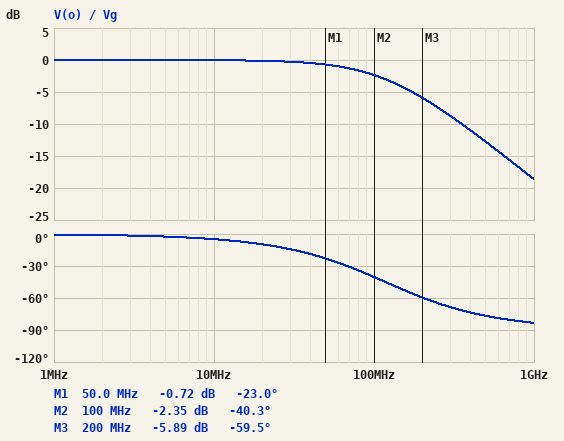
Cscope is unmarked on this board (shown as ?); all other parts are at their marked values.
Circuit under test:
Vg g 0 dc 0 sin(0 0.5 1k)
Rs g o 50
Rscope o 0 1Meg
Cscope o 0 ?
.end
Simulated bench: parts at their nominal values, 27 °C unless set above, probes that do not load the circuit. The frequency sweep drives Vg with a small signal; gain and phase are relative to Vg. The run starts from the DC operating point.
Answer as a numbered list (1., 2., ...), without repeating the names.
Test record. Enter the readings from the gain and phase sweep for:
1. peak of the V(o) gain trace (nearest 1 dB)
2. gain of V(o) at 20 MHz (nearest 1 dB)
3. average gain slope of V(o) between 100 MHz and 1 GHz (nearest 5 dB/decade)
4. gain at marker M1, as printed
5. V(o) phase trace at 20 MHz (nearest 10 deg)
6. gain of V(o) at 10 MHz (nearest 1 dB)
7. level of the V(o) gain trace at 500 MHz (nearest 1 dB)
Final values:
1. 0 dB
2. 0 dB
3. -15 dB/decade
4. -0.72 dB
5. -10 deg
6. 0 dB
7. -13 dB
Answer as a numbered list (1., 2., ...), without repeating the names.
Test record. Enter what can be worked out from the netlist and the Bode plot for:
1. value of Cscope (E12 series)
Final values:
1. 27 pF
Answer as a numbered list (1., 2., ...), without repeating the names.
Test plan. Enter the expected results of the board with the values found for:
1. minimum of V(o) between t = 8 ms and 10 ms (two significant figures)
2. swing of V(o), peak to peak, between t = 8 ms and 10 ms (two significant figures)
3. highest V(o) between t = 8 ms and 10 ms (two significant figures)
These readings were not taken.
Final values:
1. -500 mV
2. 1.0 V
3. 500 mV
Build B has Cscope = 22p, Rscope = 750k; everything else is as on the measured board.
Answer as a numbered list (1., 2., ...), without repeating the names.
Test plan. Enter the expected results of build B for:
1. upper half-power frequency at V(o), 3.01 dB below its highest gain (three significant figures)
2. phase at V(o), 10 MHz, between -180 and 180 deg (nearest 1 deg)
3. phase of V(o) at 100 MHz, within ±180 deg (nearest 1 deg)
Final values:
1. 145 MHz
2. -4 deg
3. -35 deg
